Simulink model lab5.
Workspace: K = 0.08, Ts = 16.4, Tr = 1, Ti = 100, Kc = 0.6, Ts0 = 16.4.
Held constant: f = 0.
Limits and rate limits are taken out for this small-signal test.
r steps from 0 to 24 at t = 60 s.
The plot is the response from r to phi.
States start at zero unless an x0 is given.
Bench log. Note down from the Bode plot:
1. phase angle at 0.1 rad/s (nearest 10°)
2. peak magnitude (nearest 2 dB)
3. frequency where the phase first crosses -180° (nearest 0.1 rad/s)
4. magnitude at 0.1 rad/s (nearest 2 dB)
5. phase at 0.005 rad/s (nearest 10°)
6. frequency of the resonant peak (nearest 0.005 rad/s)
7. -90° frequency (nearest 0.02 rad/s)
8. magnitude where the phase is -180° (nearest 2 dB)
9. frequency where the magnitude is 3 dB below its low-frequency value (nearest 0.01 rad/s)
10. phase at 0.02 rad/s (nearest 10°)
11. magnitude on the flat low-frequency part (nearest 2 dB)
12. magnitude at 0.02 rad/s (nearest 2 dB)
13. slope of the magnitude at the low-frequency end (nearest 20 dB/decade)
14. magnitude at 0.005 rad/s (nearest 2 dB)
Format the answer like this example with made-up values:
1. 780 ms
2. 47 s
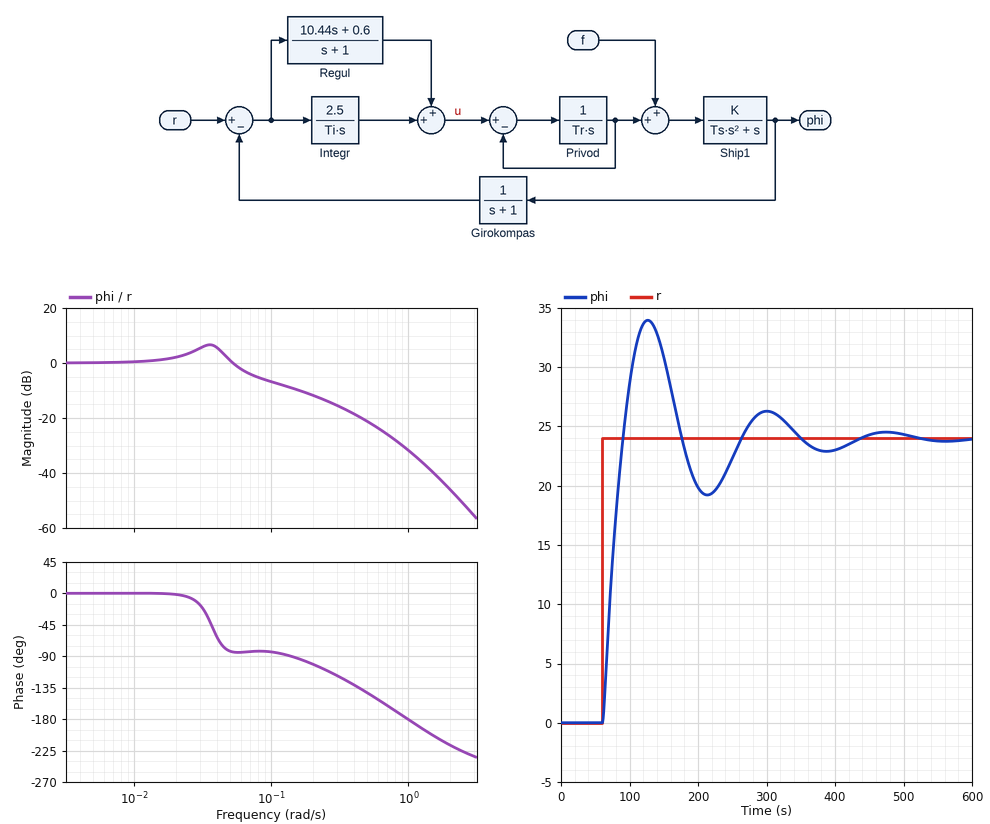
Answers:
1. -80°
2. 6 dB
3. 1.0 rad/s
4. -6 dB
5. 0°
6. 0.035 rad/s
7. 0.14 rad/s
8. -32 dB
9. 0.06 rad/s
10. 0°
11. 0 dB
12. 2 dB
13. 0 dB/decade
14. 0 dB
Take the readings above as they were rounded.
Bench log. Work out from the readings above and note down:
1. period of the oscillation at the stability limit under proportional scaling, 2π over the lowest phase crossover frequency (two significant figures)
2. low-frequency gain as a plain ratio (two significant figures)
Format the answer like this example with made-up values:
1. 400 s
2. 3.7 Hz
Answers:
1. 6.3 s
2. 1.0
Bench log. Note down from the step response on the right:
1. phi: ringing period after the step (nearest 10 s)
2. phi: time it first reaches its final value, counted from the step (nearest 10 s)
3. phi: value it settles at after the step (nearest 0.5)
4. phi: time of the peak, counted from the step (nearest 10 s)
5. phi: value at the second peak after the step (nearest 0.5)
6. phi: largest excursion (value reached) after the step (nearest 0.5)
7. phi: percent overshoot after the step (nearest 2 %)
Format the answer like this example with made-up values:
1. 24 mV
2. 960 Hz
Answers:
1. 170 s
2. 30 s
3. 24.0
4. 70 s
5. 26.5
6. 34.0
7. 42 %
